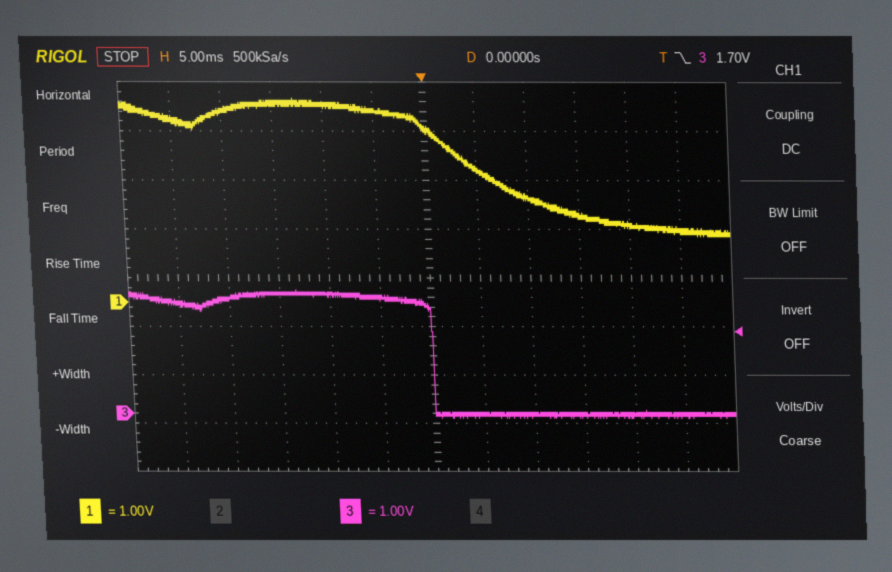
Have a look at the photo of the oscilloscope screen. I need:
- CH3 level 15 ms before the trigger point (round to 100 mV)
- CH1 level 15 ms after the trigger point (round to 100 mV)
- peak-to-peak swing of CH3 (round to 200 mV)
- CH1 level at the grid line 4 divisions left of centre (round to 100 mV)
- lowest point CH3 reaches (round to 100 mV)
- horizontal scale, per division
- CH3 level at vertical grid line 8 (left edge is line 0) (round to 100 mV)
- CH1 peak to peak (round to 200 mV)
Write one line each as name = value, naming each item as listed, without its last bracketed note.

CH3 level 15 ms before the trigger point = 2.5 V
CH1 level 15 ms after the trigger point = 1.8 V
peak-to-peak swing of CH3 = 2.6 V
CH1 level at the grid line 4 divisions left of centre = 3.9 V
lowest point CH3 reaches = -100 mV
horizontal scale, per division = 5 ms
CH3 level at vertical grid line 8 (left edge is line 0) = 0.0 V
CH1 peak to peak = 2.8 V
